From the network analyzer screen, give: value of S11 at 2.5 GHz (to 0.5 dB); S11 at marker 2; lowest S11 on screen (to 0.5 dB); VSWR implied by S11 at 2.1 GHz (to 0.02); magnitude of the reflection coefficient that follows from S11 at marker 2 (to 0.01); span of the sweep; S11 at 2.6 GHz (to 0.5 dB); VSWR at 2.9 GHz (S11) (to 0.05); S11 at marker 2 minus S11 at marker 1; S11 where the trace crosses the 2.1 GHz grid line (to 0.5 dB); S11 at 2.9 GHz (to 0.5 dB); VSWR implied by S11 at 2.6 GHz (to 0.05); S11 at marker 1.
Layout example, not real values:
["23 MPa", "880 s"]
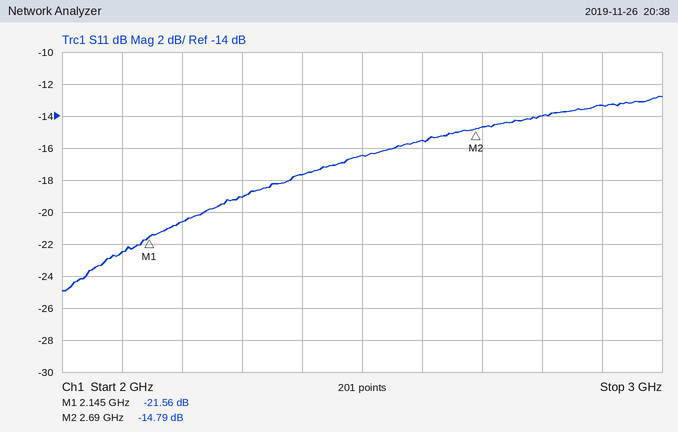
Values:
["-16.5 dB", "-14.79 dB", "-25.0 dB", "1.16", "0.18", "1 GHz", "-15.5 dB", "1.55", "6.77 dB", "-22.5 dB", "-13.5 dB", "1.40", "-21.56 dB"]
